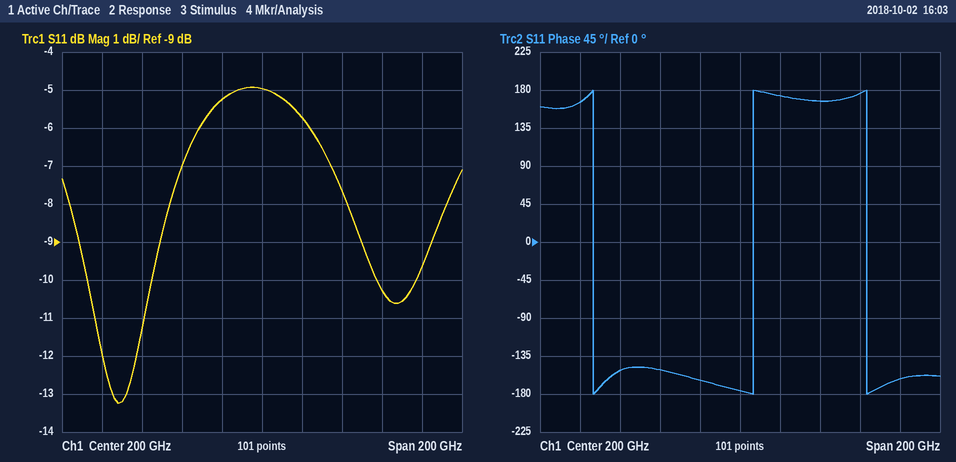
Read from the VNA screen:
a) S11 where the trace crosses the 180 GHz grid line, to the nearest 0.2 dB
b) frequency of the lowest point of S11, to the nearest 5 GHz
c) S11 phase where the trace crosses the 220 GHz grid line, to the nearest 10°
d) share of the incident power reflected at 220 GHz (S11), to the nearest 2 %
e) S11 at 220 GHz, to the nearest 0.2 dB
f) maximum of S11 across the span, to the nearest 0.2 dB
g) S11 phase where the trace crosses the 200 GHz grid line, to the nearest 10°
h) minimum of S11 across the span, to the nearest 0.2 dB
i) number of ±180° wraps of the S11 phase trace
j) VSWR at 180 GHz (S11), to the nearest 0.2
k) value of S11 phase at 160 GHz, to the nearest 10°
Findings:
-5.2 dB
130 GHz
170°
26 %
-5.8 dB
-5.0 dB
-180°
-13.2 dB
3
3.4
-150°
